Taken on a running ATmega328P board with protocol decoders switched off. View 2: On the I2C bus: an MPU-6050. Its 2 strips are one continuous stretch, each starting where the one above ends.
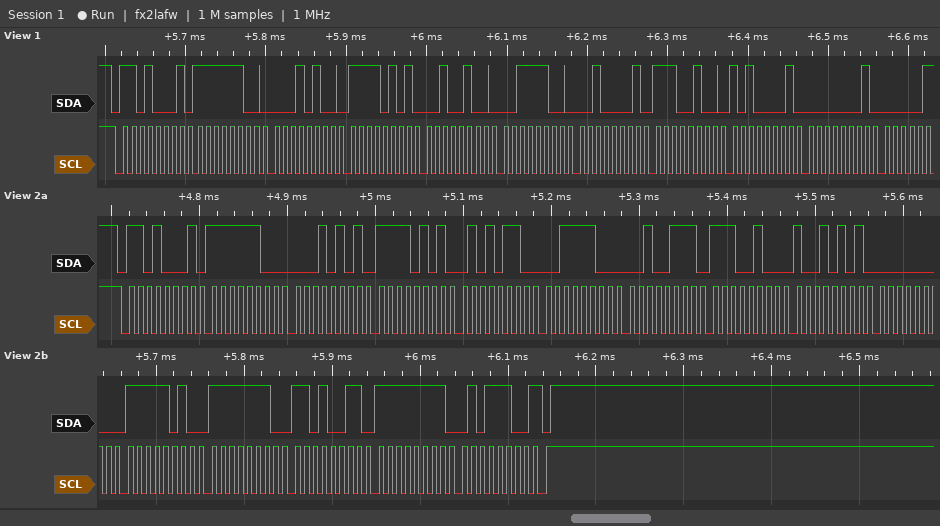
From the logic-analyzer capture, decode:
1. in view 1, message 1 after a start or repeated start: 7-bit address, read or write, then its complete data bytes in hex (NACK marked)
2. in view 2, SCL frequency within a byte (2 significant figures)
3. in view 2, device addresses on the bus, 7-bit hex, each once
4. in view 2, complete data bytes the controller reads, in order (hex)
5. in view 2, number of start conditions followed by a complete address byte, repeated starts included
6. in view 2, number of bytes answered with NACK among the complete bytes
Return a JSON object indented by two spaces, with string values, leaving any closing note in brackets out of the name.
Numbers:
{
  "in view 1, message 1 after a start or repeated start: 7-bit address, read or write, then its complete data bytes in hex": "0x68 read: FC 14 F5 24 3C 21 E4 A1 01",
  "in view 2, SCL frequency within a byte": "100 kHz",
  "in view 2, device addresses on the bus, 7-bit hex, each once": "0x68",
  "in view 2, complete data bytes the controller reads, in order": "FC 15 F5 56 3C 27 E4 95 00 FA FE D3 FF 5C",
  "in view 2, number of start conditions followed by a complete address byte, repeated starts included": "1",
  "in view 2, number of bytes answered with NACK among the complete bytes": "1"
}
